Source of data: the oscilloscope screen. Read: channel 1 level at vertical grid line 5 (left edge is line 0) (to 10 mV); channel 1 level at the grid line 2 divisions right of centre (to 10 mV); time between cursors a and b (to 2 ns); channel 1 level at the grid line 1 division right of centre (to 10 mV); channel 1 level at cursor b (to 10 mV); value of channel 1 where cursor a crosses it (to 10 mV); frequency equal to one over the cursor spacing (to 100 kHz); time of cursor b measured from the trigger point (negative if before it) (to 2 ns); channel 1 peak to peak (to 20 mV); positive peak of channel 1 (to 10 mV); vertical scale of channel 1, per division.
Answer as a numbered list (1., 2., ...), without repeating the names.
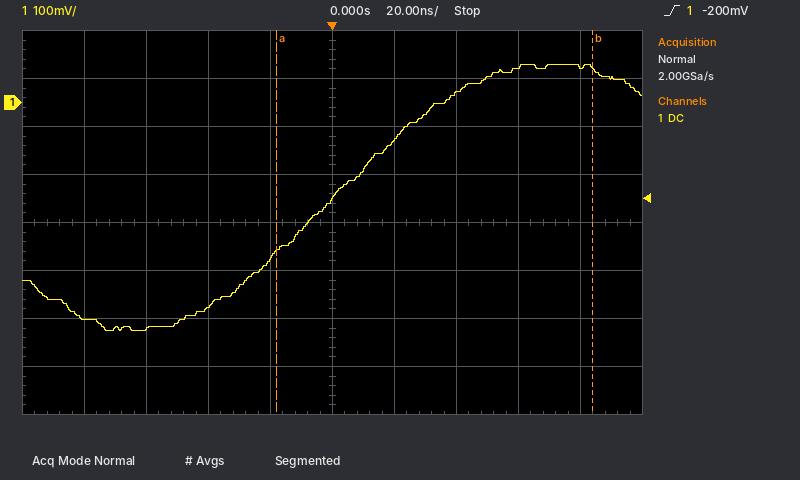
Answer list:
1. -200 mV
2. 20 mV
3. 102 ns
4. -80 mV
5. 70 mV
6. -310 mV
7. 9.8 MHz
8. +84 ns
9. 560 mV
10. 80 mV
11. 100 mV
